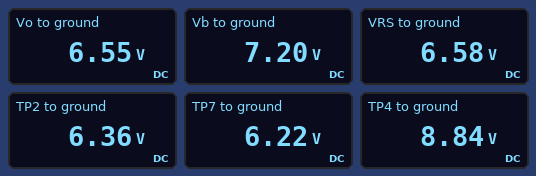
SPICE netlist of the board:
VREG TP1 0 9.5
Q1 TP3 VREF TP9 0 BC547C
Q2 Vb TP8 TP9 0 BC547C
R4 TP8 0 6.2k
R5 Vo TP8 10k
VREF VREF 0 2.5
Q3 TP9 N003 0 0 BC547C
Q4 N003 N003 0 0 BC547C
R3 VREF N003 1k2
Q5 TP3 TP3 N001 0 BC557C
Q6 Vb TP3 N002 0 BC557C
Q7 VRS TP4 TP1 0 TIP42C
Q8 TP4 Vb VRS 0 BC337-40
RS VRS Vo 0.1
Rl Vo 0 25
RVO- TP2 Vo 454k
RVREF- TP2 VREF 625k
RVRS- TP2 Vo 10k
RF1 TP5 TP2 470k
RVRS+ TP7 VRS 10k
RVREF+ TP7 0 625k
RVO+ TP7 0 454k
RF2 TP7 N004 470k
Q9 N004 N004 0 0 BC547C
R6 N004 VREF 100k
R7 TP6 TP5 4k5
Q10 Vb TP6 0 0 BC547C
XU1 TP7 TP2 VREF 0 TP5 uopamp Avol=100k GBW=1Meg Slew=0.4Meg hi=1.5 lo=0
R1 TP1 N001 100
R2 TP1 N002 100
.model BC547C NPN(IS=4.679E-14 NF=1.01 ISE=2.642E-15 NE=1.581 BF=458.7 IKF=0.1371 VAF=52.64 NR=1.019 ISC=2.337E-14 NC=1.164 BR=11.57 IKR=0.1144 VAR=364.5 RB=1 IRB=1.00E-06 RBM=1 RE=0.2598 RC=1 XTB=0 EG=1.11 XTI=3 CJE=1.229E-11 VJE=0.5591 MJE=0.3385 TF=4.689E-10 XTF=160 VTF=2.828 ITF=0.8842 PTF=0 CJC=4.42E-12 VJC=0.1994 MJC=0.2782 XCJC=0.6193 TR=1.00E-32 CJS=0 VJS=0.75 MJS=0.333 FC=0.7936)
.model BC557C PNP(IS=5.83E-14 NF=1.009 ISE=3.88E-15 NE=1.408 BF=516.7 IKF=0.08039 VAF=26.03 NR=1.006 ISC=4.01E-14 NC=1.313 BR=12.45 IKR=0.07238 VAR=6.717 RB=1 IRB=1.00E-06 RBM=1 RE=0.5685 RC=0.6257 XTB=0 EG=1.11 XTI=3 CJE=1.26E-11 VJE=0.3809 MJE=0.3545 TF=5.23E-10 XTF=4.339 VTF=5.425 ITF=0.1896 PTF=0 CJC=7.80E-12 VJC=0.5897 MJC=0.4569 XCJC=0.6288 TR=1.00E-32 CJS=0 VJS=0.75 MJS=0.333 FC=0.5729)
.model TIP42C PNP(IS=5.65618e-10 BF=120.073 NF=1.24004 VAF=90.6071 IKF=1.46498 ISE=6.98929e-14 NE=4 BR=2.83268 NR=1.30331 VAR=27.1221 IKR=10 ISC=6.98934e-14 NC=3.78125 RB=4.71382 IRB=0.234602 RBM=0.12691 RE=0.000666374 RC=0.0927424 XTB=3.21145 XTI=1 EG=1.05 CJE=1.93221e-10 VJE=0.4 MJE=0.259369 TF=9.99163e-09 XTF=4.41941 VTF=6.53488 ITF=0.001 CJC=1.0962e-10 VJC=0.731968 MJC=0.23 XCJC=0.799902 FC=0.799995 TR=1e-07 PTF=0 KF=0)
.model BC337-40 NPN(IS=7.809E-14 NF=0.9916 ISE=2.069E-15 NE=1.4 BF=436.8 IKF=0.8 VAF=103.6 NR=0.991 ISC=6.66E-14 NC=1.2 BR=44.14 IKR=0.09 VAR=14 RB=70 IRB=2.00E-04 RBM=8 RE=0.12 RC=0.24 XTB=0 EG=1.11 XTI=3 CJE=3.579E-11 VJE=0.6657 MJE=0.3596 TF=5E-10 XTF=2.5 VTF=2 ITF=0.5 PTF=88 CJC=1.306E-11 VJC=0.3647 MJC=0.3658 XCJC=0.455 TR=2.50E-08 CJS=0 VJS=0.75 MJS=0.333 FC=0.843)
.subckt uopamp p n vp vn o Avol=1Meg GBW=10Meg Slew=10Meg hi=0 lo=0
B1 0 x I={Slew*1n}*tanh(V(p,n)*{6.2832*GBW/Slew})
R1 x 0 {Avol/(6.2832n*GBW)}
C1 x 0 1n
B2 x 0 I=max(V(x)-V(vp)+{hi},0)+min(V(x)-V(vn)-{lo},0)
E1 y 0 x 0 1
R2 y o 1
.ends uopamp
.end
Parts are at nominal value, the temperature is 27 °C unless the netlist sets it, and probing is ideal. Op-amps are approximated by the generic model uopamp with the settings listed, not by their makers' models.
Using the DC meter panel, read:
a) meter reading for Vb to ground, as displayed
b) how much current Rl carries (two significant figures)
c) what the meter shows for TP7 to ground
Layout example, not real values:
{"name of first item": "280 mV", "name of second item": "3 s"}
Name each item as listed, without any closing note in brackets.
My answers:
{"meter reading for Vb to ground, as displayed": "7.20 V", "how much current Rl carries": "260 mA", "what the meter shows for TP7 to ground": "6.22 V"}
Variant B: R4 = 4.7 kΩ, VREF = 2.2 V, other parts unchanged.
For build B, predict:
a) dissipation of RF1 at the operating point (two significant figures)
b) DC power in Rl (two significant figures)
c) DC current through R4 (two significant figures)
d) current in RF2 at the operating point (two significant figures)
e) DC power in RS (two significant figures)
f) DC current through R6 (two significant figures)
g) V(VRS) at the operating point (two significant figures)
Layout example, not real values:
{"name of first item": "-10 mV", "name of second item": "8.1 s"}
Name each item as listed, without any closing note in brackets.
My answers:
{"dissipation of RF1 at the operating point": "95 µW", "DC power in Rl": "1.9 W", "DC current through R4": "470 µA", "current in RF2 at the operating point": "13 µA", "DC power in RS": "7.6 mW", "DC current through R6": "17 µA", "V(VRS) at the operating point": "6.9 V"}
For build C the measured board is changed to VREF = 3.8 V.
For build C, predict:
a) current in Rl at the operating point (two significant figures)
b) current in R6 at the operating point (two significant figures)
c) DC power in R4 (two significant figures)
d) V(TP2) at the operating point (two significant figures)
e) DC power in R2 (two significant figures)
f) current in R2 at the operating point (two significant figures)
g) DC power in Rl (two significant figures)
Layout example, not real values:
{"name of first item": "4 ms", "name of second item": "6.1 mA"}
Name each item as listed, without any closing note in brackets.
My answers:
{"current in Rl at the operating point": "350 mA", "current in R6 at the operating point": "33 µA", "DC power in R4": "1.8 mW", "V(TP2) at the operating point": "8.5 V", "DC power in R2": "120 µW", "current in R2 at the operating point": "1.1 mA", "DC power in Rl": "3.0 W"}
